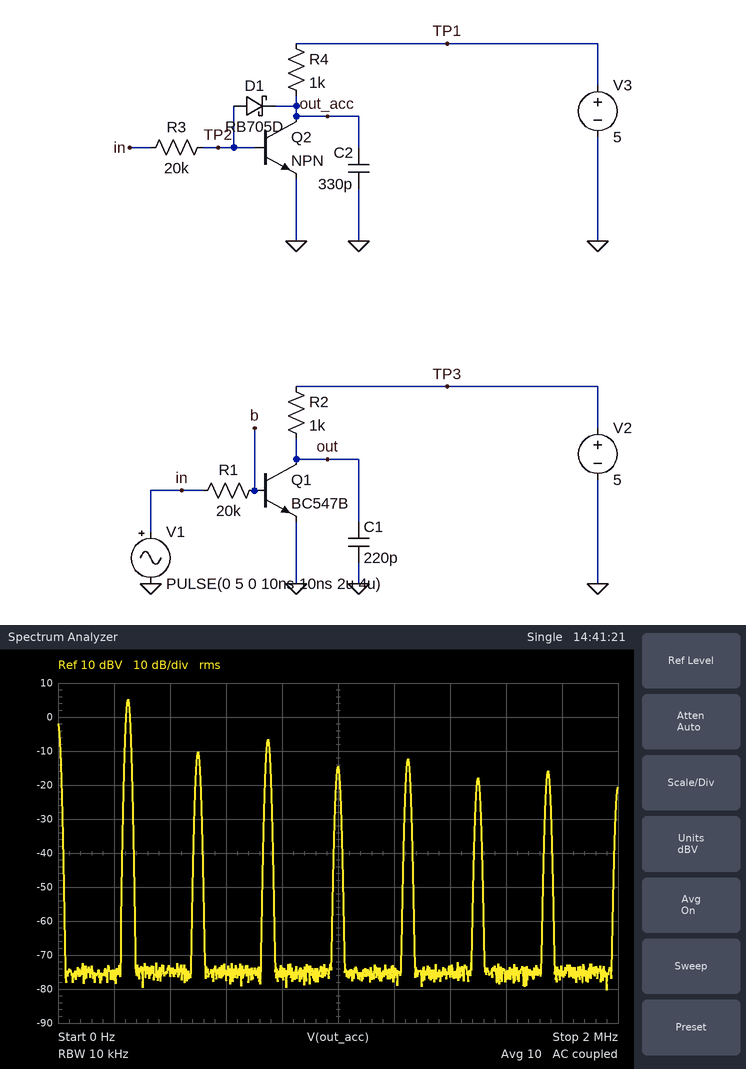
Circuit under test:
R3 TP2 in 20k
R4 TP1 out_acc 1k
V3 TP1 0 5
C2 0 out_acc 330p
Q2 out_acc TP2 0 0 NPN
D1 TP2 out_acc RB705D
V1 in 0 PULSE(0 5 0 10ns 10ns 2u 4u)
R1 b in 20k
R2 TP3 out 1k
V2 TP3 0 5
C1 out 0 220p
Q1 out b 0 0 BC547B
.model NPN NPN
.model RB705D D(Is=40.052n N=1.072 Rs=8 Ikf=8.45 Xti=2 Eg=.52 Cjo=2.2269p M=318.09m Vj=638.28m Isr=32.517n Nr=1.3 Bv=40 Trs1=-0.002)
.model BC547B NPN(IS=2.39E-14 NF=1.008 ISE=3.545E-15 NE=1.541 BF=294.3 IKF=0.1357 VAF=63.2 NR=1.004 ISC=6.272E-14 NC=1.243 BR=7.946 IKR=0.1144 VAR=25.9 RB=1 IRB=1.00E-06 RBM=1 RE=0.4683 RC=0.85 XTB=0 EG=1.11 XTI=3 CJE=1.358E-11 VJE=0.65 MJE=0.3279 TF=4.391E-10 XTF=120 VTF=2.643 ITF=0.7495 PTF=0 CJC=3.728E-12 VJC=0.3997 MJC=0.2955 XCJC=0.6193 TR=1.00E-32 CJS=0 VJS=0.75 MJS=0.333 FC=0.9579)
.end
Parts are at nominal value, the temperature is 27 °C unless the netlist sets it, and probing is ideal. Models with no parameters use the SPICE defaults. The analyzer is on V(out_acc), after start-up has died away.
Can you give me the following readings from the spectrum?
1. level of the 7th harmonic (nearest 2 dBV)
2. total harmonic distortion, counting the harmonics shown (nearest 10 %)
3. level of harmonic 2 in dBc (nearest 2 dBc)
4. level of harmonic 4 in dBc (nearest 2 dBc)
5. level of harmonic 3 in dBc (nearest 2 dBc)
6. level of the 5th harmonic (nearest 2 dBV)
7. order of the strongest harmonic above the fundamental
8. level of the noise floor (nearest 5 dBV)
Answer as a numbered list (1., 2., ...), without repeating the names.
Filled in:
1. -16 dBV
2. 40 %
3. -16 dBc
4. -20 dBc
5. -12 dBc
6. -12 dBV
7. 3
8. -75 dBV
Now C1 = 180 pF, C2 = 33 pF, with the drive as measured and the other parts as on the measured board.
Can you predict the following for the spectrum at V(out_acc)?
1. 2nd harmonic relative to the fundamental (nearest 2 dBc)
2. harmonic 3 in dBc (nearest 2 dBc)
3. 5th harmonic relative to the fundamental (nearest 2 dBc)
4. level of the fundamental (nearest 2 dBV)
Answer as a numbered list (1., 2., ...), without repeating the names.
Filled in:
1. -26 dBc
2. -10 dBc
3. -14 dBc
4. 6 dBV
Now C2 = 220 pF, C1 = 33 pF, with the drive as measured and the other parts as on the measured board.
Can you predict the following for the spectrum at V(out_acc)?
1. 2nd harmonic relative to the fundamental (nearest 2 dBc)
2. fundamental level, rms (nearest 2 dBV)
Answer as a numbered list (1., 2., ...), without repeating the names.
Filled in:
1. -18 dBc
2. 6 dBV
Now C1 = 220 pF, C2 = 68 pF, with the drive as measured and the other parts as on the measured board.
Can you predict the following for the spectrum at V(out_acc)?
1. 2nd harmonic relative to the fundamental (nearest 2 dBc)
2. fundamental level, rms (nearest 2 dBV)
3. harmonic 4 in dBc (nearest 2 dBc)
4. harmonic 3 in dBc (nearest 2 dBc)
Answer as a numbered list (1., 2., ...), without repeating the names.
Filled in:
1. -24 dBc
2. 6 dBV
3. -26 dBc
4. -10 dBc
